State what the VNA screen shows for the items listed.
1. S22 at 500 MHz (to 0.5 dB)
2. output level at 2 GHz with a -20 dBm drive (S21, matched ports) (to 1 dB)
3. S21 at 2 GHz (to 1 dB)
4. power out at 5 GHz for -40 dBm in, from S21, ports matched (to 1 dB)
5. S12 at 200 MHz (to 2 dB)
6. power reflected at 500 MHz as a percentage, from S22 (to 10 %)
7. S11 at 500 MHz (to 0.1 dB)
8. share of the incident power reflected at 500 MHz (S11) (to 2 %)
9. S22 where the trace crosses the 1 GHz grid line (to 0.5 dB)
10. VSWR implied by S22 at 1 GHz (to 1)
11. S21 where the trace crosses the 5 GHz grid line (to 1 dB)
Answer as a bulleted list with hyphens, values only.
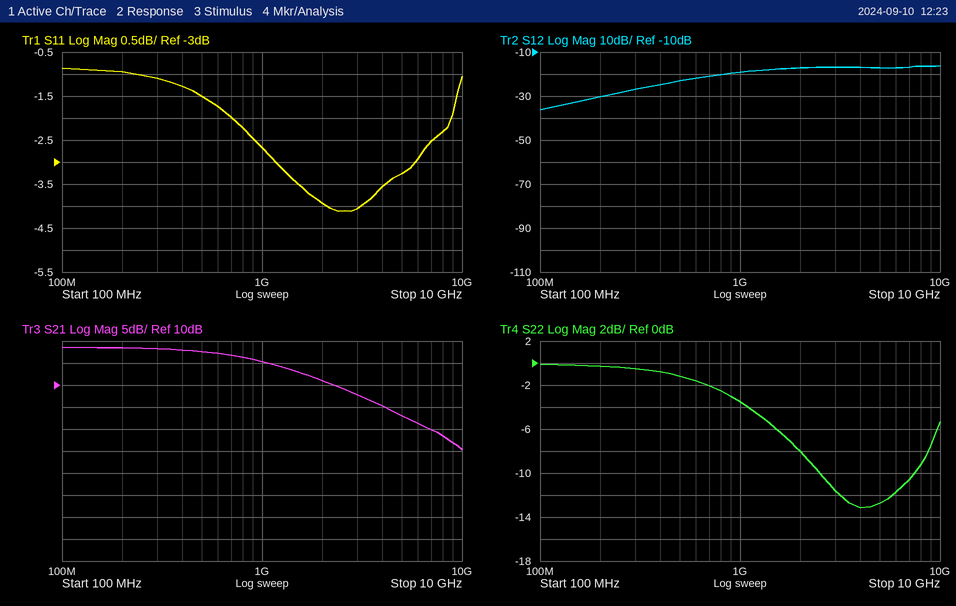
- -1.0 dB
- -9 dBm
- 11 dB
- -37 dBm
- -30 dB
- 80 %
- -1.5 dB
- 70 %
- -3.5 dB
- 5
- 3 dB
